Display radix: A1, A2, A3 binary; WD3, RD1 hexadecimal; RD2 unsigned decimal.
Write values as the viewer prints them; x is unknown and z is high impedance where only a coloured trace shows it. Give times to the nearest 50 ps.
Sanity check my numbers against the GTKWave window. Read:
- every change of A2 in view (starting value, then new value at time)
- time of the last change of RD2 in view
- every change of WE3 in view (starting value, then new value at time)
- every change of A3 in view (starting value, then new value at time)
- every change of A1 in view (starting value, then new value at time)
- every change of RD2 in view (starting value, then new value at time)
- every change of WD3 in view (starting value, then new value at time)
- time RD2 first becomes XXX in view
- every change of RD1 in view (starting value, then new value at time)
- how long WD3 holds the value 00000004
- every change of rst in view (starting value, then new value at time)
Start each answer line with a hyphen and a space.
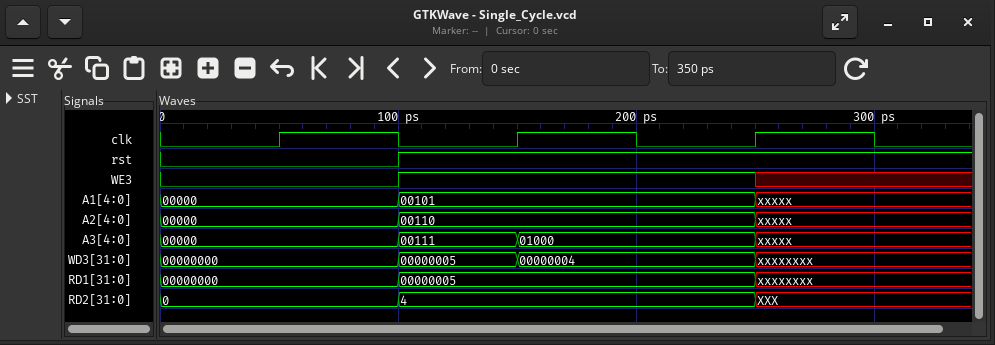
- 00000, 00110 at 100 ps, xxxxx at 250 ps
- 250 ps
- 0, 1 at 100 ps, x at 250 ps
- 00000, 00111 at 100 ps, 01000 at 150 ps, xxxxx at 250 ps
- 00000, 00101 at 100 ps, xxxxx at 250 ps
- 0, 4 at 100 ps, XXX at 250 ps
- 00000000, 00000005 at 100 ps, 00000004 at 150 ps, xxxxxxxx at 250 ps
- 250 ps
- 00000000, 00000005 at 100 ps, xxxxxxxx at 250 ps
- 100 ps
- 0, 1 at 100 ps
